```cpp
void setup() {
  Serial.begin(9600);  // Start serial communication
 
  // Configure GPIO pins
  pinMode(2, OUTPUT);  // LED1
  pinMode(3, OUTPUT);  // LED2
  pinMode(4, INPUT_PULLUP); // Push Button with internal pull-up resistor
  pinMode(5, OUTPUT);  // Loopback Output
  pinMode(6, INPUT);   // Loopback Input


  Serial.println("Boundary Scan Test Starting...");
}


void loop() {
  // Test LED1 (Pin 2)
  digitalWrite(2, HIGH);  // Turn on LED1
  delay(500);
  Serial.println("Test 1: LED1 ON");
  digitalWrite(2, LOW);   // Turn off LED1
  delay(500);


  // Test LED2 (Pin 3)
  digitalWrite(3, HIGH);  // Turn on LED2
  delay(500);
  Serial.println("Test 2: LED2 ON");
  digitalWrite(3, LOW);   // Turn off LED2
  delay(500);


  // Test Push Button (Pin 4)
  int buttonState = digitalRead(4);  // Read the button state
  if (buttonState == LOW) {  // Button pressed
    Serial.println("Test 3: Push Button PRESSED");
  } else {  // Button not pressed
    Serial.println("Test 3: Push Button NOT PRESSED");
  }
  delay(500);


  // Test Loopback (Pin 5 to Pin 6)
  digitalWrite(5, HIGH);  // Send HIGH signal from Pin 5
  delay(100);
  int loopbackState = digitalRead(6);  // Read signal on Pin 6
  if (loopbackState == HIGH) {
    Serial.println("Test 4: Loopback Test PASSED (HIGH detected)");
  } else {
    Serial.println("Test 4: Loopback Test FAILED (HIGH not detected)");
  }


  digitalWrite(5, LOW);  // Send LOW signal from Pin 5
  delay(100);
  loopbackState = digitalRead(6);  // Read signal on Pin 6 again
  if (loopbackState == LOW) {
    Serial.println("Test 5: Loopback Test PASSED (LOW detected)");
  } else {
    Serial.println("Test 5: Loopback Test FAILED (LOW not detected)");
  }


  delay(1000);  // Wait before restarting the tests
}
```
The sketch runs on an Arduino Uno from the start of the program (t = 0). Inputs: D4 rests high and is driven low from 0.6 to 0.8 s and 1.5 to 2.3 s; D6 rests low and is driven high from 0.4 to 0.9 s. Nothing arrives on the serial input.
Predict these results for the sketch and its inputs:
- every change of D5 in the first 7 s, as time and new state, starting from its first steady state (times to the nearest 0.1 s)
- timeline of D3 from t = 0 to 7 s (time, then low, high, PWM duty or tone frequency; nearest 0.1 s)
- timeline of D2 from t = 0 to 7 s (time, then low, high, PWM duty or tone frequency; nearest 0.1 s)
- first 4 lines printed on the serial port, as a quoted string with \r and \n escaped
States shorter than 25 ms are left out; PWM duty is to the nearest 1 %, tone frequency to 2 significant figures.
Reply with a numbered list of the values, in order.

1. 0 s low; 2.5 s high; 2.6 s low; 6.2 s high; 6.3 s low
2. 0 s low; 1 s high; 1.5 s low; 4.7 s high; 5.2 s low
3. 0 s high; 0.5 s low; 3.7 s high; 4.2 s low
4. "Boundary Scan Test Starting...\r\nTest 1: LED1 ON\r\nTest 2: LED2 ON\r\nTest 3: Push Button PRESSED\r\n"
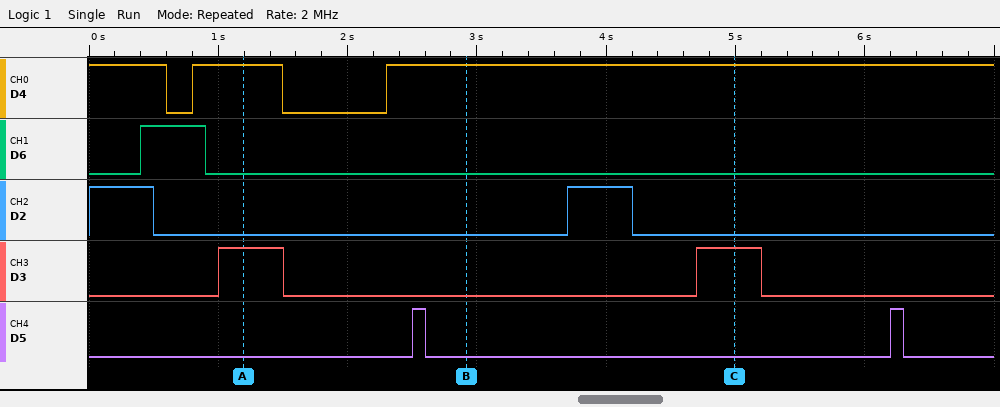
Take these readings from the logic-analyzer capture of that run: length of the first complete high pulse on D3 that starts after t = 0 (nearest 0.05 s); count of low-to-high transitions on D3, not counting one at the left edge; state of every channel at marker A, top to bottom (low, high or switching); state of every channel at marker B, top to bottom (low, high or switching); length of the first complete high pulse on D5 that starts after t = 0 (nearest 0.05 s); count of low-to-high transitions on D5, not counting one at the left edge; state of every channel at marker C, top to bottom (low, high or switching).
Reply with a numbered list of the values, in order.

1. 0.50 s
2. 2
3. D4 high, D6 low, D2 low, D3 high, D5 low
4. D4 high, D6 low, D2 low, D3 low, D5 low
5. 0.10 s
6. 2
7. D4 high, D6 low, D2 low, D3 high, D5 low
